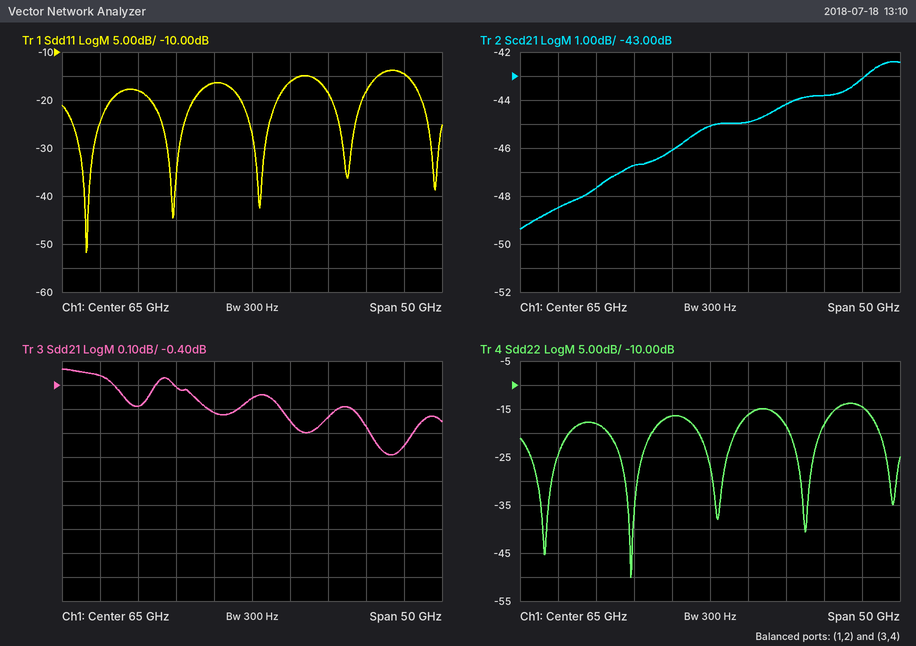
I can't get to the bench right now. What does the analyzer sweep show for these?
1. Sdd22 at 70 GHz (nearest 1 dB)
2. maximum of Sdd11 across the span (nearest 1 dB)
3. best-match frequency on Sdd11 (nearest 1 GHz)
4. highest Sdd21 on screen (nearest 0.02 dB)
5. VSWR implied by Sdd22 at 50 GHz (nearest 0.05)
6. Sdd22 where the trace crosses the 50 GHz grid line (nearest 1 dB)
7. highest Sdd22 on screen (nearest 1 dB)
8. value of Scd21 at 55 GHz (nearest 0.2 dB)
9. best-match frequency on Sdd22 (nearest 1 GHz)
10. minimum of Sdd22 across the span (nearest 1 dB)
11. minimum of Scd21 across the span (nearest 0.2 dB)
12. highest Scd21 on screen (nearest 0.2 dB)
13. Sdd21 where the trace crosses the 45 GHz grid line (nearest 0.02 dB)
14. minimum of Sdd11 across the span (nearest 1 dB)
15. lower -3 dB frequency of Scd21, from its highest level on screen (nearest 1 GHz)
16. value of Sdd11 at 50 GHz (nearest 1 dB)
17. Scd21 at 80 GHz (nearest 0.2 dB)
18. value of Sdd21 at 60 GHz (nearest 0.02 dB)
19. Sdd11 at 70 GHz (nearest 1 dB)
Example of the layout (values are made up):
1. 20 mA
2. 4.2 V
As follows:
1. -16 dB
2. -14 dB
3. 43 GHz
4. -0.34 dB
5. 1.30
6. -18 dB
7. -14 dB
8. -46.8 dB
9. 55 GHz
10. -50 dB
11. -49.4 dB
12. -42.4 dB
13. -0.36 dB
14. -52 dB
15. 63 GHz
16. -18 dB
17. -43.8 dB
18. -0.52 dB
19. -16 dB
